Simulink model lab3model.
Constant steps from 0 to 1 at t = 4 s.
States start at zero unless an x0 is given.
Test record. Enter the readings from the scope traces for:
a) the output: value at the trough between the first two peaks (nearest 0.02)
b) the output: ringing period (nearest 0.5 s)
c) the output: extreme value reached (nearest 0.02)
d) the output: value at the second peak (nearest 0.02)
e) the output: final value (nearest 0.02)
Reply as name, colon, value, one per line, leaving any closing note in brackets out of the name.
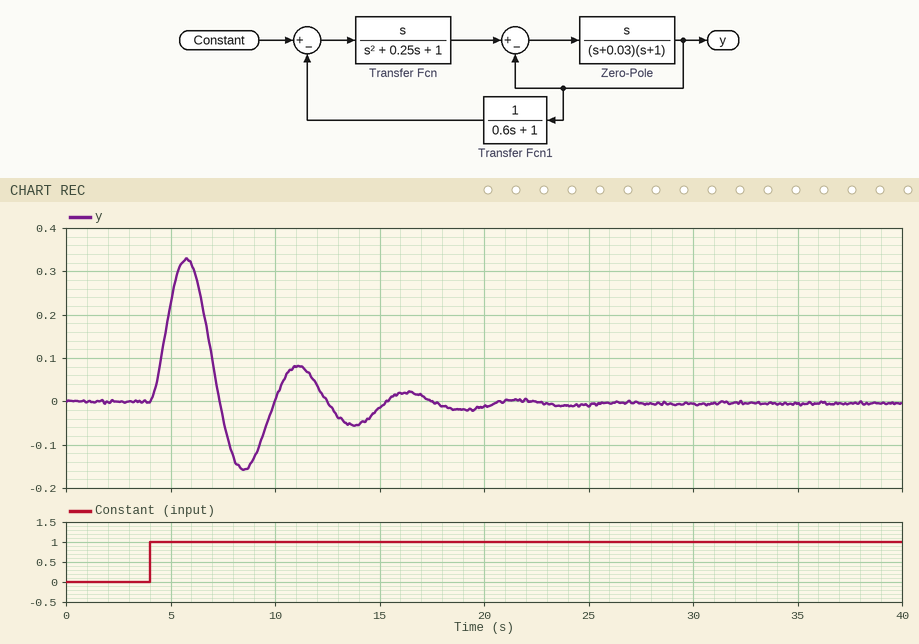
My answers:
the output: value at the trough between the first two peaks: -0.16
the output: ringing period: 5.5 s
the output: extreme value reached: 0.32
the output: value at the second peak: 0.08
the output: final value: 0.00
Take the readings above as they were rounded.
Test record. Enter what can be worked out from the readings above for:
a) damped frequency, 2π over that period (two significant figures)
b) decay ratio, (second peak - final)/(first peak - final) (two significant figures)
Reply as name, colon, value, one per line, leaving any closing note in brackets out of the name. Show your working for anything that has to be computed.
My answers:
damped frequency, 2π over that period: 2π / 5.5 = 1.1 rad/s
decay ratio, (second peak - final)/(first peak - final): (0.08 - 0) / (0.32 - 0) = 0.25
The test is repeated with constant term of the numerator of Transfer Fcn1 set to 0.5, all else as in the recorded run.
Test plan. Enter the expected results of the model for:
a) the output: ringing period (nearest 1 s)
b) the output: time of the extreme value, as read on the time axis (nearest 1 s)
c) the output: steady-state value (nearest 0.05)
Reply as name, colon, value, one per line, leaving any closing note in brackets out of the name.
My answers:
the output: ringing period: 6 s
the output: time of the extreme value, as read on the time axis: 6 s
the output: steady-state value: 0.00
